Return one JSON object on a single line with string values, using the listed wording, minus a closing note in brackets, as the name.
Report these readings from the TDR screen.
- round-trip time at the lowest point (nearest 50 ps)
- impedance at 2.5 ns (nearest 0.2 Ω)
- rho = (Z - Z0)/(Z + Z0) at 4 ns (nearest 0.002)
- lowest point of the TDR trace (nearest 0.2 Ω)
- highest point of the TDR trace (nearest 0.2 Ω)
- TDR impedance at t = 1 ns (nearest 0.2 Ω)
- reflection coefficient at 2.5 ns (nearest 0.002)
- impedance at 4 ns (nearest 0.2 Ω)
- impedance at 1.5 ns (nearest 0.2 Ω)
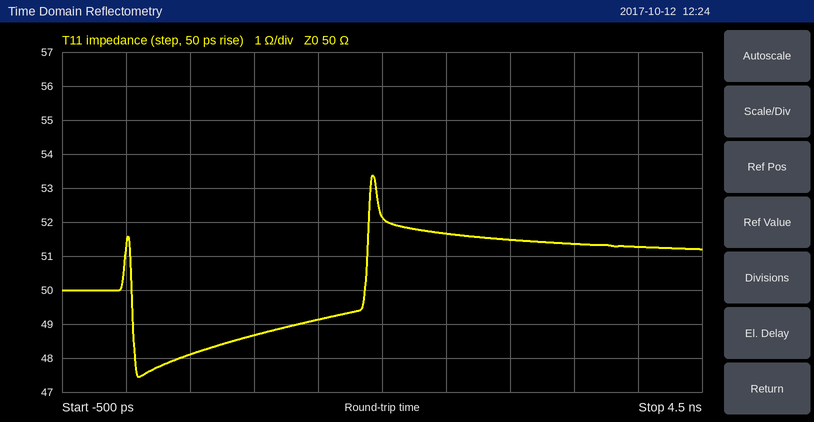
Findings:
{"round-trip time at the lowest point": "100 ps", "impedance at 2.5 ns": "51.6 Ω", "rho = (Z - Z0)/(Z + Z0) at 4 ns": "+0.012", "lowest point of the TDR trace": "47.4 Ω", "highest point of the TDR trace": "53.4 Ω", "TDR impedance at t = 1 ns": "48.6 Ω", "reflection coefficient at 2.5 ns": "+0.016", "impedance at 4 ns": "51.2 Ω", "impedance at 1.5 ns": "49.2 Ω"}
